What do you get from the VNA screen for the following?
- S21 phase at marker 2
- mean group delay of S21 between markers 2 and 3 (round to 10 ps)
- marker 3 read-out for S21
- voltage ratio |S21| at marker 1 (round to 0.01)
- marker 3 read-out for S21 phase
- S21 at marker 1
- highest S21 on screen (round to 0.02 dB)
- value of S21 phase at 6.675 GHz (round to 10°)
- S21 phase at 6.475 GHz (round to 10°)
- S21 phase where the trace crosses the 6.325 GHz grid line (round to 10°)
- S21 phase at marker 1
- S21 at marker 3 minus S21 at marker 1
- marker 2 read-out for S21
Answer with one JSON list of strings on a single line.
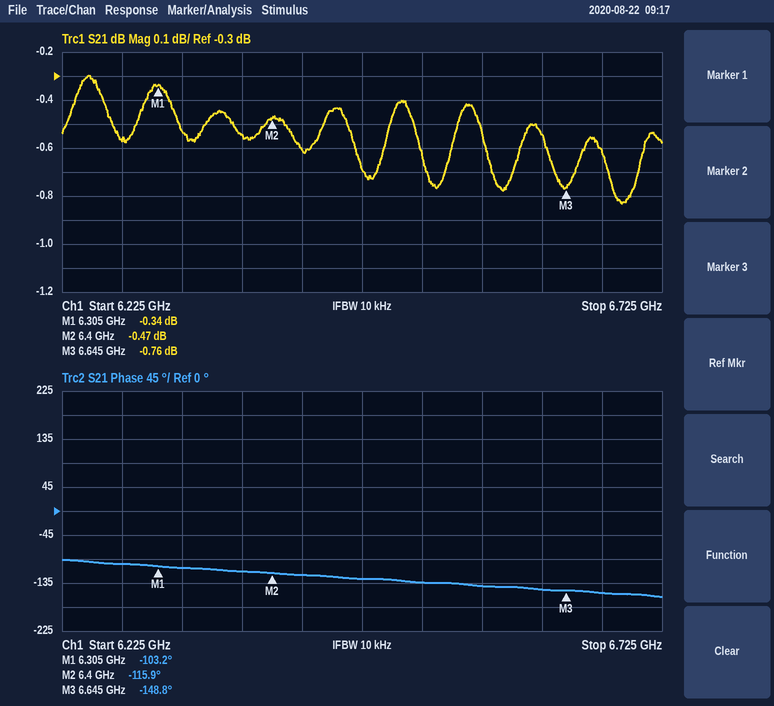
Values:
["-115.9°", "370 ps", "-0.76 dB", "0.96", "-148.8°", "-0.34 dB", "-0.30 dB", "-150°", "-130°", "-110°", "-103.2°", "-0.42 dB", "-0.47 dB"]
